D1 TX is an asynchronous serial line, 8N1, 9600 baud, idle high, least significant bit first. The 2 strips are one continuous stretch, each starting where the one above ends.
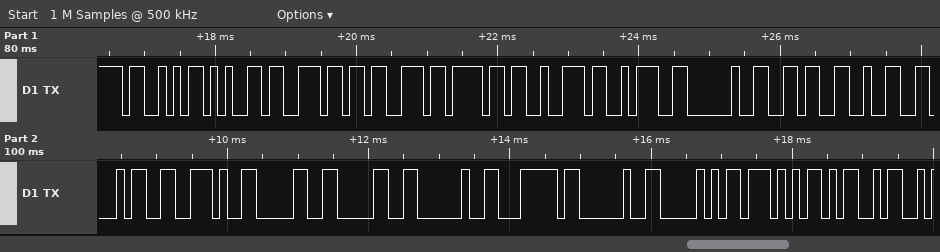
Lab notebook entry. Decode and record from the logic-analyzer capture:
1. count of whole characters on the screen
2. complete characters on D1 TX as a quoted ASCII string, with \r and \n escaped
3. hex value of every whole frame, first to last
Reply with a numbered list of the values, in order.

1. 20
2. "Sensor: 624.00 | PWM"
3. 53 65 6E 73 6F 72 3A 20 36 32 34 2E 30 30 20 7C 20 50 57 4D
